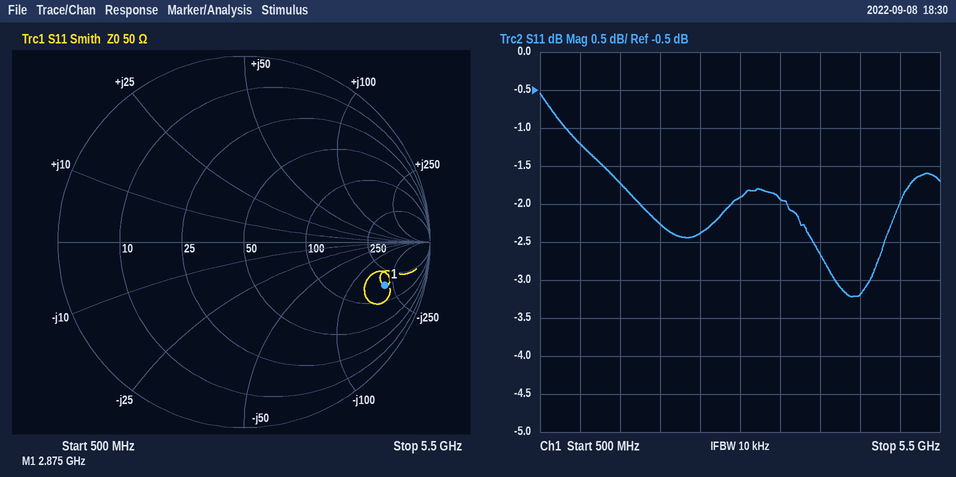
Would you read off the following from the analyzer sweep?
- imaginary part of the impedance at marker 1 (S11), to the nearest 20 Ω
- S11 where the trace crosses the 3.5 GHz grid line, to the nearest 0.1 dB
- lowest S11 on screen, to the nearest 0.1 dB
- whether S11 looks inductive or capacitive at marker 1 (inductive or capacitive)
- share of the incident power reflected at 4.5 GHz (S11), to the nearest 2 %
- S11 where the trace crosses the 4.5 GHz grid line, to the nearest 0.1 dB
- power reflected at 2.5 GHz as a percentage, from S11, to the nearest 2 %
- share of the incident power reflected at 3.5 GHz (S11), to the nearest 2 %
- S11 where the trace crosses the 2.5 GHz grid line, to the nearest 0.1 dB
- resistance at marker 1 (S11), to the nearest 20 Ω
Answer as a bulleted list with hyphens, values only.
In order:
- -200 Ω
- -1.9 dB
- -3.2 dB
- capacitive
- 48 %
- -3.2 dB
- 58 %
- 64 %
- -2.4 dB
- 160 Ω
